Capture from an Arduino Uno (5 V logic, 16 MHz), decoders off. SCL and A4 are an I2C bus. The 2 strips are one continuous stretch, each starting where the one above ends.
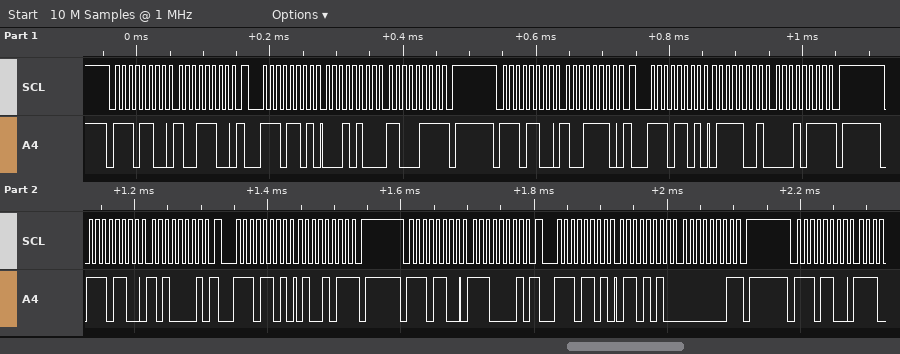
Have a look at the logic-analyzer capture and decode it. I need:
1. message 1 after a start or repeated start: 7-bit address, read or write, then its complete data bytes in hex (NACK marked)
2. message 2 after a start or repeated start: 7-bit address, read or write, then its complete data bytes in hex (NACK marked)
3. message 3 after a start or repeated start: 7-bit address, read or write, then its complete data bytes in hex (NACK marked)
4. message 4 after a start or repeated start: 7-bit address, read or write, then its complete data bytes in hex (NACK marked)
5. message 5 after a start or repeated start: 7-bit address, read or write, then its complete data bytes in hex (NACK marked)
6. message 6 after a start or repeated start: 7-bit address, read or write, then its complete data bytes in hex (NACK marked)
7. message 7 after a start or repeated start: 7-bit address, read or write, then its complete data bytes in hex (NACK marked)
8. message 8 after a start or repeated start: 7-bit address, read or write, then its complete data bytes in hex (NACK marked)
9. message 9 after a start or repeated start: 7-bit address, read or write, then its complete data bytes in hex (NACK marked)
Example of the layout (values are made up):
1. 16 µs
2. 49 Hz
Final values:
1. 0x76 write: 9C
2. 0x76 read: 14 C7 NACK
3. 0x76 write: 9E
4. 0x76 read: 79 17 NACK
5. 0x76 write: A1
6. 0x76 read: 4B NACK
7. 0x76 write: E1
8. 0x76 read: 6A 01 NACK
9. 0x76 write
